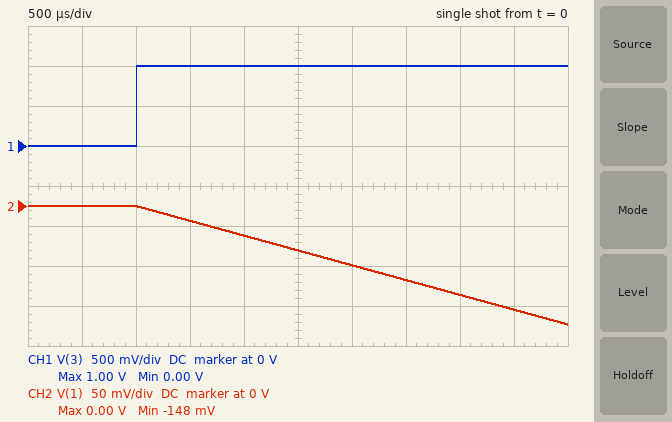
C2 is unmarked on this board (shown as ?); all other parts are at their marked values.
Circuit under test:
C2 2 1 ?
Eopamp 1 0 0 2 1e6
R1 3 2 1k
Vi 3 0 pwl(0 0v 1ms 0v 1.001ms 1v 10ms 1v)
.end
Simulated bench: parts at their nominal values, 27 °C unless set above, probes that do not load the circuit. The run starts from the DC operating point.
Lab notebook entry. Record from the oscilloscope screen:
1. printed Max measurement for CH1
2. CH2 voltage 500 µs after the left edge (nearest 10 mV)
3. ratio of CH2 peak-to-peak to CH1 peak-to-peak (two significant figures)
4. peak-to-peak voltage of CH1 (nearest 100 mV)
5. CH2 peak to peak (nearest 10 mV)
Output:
1.00 V
0 V
0.15
1.0 V
150 mV
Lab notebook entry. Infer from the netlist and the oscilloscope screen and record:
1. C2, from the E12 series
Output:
27 µF
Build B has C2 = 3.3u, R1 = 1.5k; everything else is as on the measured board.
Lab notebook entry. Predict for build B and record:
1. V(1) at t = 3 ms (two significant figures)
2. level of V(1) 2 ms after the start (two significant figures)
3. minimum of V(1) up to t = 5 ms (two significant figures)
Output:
-400 mV
-200 mV
-810 mV
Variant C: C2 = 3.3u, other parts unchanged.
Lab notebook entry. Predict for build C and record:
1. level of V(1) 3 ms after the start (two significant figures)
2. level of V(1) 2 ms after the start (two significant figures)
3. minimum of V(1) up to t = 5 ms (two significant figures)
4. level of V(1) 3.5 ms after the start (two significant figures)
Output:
-610 mV
-300 mV
-1.2 V
-760 mV
